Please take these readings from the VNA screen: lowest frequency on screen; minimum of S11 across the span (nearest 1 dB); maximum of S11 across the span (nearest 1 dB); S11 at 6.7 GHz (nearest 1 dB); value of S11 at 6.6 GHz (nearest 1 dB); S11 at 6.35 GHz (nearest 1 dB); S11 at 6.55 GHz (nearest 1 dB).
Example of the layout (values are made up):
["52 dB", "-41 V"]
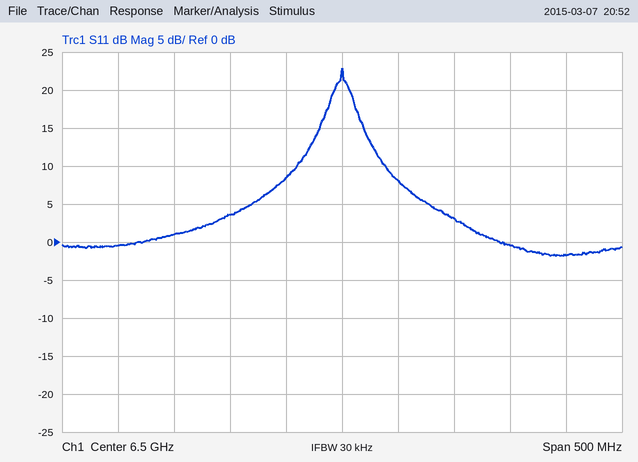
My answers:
["6.25 GHz", "-2 dB", "23 dB", "-2 dB", "3 dB", "1 dB", "8 dB"]
